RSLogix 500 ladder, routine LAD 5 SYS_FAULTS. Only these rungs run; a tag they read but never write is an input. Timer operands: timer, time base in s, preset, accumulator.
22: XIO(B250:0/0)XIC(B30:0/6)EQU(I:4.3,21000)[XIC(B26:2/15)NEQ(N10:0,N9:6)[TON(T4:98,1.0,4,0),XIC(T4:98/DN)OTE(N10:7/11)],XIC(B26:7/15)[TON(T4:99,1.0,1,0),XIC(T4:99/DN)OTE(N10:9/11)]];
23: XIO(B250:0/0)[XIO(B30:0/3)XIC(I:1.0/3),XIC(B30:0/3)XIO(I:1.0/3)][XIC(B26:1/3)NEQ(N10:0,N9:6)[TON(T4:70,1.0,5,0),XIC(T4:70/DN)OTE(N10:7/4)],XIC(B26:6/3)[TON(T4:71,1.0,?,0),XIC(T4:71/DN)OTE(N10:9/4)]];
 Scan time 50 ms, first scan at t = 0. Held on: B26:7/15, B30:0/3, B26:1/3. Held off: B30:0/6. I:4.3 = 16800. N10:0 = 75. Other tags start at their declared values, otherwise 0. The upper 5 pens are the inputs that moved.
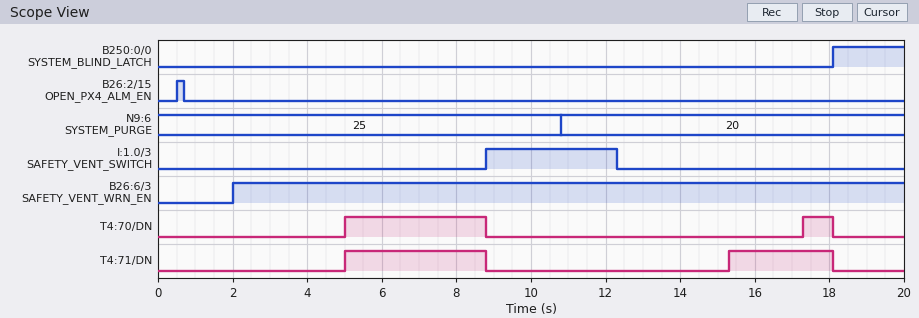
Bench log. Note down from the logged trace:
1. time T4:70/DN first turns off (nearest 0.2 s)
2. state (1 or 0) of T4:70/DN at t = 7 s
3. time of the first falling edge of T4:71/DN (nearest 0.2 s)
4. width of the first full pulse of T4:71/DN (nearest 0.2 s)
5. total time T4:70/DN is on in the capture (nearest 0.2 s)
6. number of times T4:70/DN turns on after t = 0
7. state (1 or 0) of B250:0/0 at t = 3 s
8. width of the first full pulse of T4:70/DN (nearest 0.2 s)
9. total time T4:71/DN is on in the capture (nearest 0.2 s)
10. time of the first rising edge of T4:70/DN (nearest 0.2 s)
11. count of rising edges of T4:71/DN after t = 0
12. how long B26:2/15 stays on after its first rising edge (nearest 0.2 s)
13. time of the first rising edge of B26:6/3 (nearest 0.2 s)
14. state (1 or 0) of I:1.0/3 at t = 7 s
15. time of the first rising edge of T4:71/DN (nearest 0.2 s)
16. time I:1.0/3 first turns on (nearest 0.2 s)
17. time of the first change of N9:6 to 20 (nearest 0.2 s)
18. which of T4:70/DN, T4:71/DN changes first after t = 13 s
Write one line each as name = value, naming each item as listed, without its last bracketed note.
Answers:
time T4:70/DN first turns off = 8.8 s
state (1 or 0) of T4:70/DN at t = 7 s = 1
time of the first falling edge of T4:71/DN = 8.8 s
width of the first full pulse of T4:71/DN = 3.8 s
total time T4:70/DN is on in the capture = 4.6 s
number of times T4:70/DN turns on after t = 0 = 2
state (1 or 0) of B250:0/0 at t = 3 s = 0
width of the first full pulse of T4:70/DN = 3.8 s
total time T4:71/DN is on in the capture = 6.6 s
time of the first rising edge of T4:70/DN = 5.0 s
count of rising edges of T4:71/DN after t = 0 = 2
how long B26:2/15 stays on after its first rising edge = 0.2 s
time of the first rising edge of B26:6/3 = 2.0 s
state (1 or 0) of I:1.0/3 at t = 7 s = 0
time of the first rising edge of T4:71/DN = 5.0 s
time I:1.0/3 first turns on = 8.8 s
time of the first change of N9:6 to 20 = 10.8 s
which of T4:70/DN, T4:71/DN changes first after t = 13 s = T4:71/DN
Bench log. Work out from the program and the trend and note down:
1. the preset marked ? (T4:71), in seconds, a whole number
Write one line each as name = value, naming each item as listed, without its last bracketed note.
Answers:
the preset marked ? (T4:71), in seconds, a whole number = 3 s
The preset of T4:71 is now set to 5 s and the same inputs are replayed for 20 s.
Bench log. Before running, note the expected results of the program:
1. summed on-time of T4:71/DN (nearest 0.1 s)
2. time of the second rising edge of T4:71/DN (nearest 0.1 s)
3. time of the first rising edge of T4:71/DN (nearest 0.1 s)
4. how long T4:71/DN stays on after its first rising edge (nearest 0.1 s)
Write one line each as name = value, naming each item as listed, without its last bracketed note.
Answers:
summed on-time of T4:71/DN = 2.6 s
time of the second rising edge of T4:71/DN = 17.3 s
time of the first rising edge of T4:71/DN = 7.0 s
how long T4:71/DN stays on after its first rising edge = 1.8 s
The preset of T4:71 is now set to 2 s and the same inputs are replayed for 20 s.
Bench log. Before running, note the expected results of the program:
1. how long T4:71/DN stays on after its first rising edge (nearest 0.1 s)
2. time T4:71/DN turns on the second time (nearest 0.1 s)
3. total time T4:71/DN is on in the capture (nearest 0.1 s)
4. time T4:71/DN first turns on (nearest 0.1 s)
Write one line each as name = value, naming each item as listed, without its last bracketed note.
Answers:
how long T4:71/DN stays on after its first rising edge = 4.8 s
time T4:71/DN turns on the second time = 14.3 s
total time T4:71/DN is on in the capture = 8.6 s
time T4:71/DN first turns on = 4.0 s
